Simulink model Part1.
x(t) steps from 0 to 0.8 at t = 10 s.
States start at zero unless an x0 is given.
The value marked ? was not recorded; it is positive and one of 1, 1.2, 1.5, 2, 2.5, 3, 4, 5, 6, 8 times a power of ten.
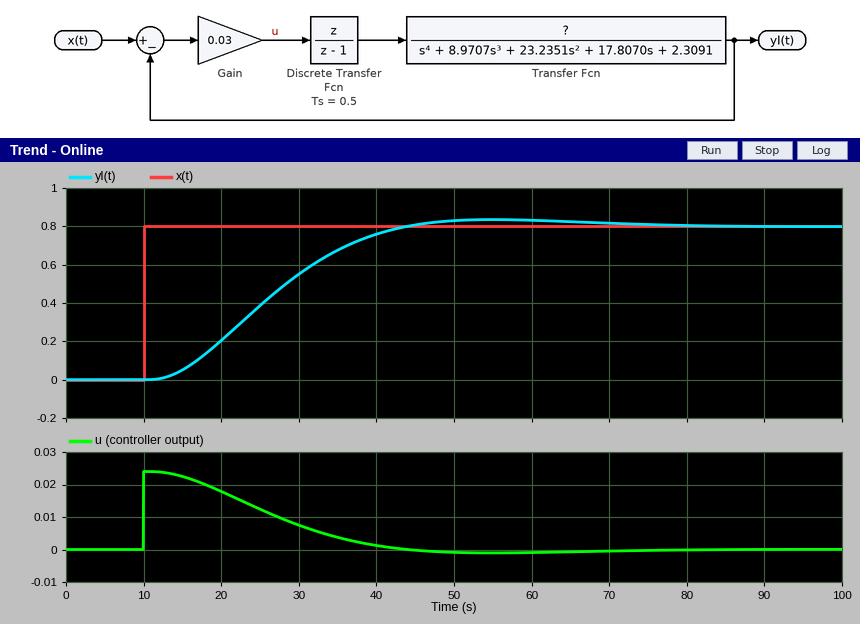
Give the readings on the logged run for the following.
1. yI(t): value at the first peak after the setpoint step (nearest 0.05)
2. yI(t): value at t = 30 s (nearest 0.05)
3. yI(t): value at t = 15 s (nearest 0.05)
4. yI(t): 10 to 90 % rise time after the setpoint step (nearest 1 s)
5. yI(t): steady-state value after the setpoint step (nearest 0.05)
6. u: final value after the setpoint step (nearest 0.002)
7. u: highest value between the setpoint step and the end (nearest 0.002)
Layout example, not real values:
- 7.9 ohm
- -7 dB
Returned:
- 0.85
- 0.55
- 0.05
- 21 s
- 0.80
- 0.000
- 0.024
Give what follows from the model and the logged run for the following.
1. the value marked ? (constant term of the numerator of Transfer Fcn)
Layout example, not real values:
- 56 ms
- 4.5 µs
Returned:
- 2.5
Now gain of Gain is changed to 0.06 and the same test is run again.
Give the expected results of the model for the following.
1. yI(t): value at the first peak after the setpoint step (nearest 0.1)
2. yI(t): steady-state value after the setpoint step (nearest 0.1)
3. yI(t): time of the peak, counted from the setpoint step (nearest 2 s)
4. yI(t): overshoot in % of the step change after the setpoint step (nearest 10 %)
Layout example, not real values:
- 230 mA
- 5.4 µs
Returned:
- 1.0
- 0.8
- 26 s
- 20 %
